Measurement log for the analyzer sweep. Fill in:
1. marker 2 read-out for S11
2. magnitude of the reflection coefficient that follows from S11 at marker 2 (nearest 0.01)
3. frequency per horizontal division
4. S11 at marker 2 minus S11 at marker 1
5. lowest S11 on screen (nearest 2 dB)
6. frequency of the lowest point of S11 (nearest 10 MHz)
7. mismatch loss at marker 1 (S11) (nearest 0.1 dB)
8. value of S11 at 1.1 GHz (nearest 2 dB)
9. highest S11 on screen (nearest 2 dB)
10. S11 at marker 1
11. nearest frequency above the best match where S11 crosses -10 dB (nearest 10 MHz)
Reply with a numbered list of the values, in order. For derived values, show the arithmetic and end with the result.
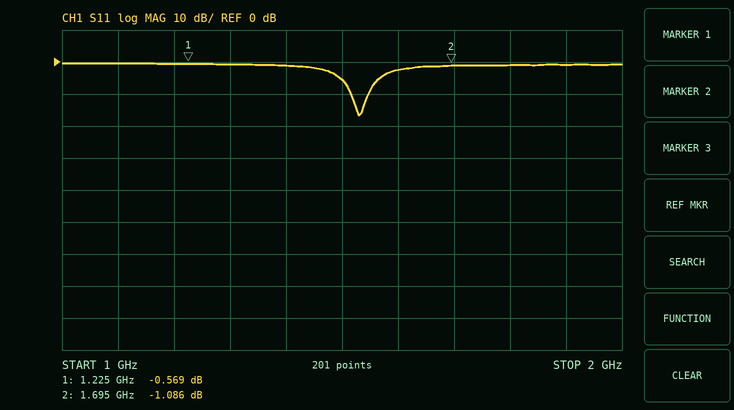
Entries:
1. -1.086 dB
2. 10^(-1.086/20) ≈ 0.88
3. 100 MHz
4. -1.086 − (-0.569) = -0.517 dB
5. -16 dB
6. 1.53 GHz
7. −10 log10(1 − 10^(-0.569/10)) ≈ 9.1 dB
8. 0 dB
9. 0 dB
10. -0.569 dB
11. 1.55 GHz
